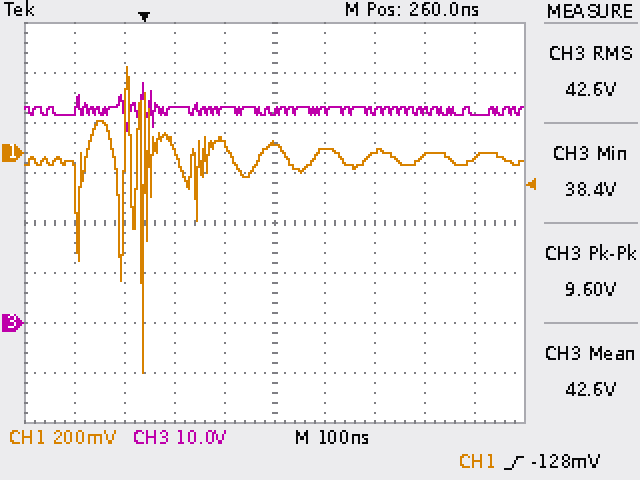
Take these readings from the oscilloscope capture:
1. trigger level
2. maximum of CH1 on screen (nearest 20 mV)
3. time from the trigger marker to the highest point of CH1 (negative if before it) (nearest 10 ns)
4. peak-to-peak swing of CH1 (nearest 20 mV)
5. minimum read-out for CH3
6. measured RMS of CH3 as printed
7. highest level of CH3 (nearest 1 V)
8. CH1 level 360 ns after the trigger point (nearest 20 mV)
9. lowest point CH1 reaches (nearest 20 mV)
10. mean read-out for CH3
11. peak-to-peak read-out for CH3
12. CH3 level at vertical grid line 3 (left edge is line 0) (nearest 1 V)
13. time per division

-128 mV
340 mV
-30 ns
1.22 V
38.4 V
42.6 V
48 V
20 mV
-880 mV
42.6 V
9.60 V
43 V
100 ns
